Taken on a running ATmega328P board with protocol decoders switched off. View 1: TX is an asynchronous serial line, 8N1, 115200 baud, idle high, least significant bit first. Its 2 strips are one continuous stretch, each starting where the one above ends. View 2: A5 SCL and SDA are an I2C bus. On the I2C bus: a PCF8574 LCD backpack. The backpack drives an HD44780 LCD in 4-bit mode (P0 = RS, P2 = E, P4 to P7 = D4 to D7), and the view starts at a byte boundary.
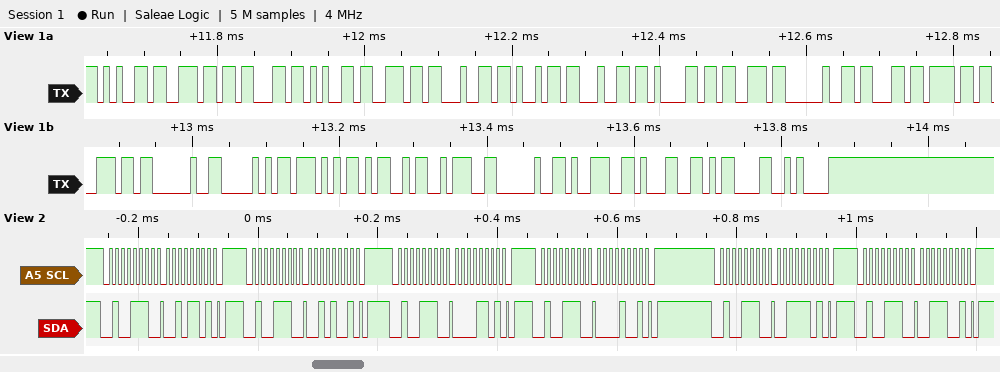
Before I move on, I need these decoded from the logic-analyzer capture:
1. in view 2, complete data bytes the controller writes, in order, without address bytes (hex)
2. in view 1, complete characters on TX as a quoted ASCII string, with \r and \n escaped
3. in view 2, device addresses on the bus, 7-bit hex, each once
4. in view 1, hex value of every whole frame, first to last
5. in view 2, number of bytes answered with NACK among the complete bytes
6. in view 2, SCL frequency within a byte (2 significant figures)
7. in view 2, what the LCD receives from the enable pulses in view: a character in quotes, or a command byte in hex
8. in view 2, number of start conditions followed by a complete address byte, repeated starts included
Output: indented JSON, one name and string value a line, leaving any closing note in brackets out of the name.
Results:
{
  "in view 2, complete data bytes the controller writes, in order, without address bytes": "2D 29 0D 09 3D 39",
  "in view 1, complete characters on TX as a quoted ASCII string, with \\r and \\n escaped": "\"encendidas con PWM: 91\\r\\n\"",
  "in view 2, device addresses on the bus, 7-bit hex, each once": "0x27",
  "in view 1, hex value of every whole frame, first to last": "65 6E 63 65 6E 64 69 64 61 73 20 63 6F 6E 20 50 57 4D 3A 20 39 31 0D 0A",
  "in view 2, number of bytes answered with NACK among the complete bytes": "0",
  "in view 2, SCL frequency within a byte": "100 kHz",
  "in view 2, what the LCD receives from the enable pulses in view: a character in quotes, or a command byte in hex": "' '",
  "in view 2, number of start conditions followed by a complete address byte, repeated starts included": "6"
}
